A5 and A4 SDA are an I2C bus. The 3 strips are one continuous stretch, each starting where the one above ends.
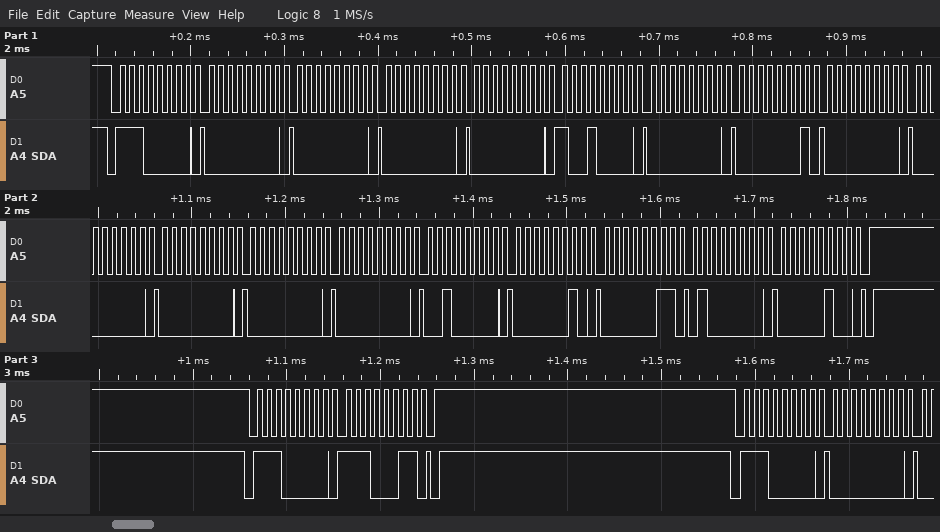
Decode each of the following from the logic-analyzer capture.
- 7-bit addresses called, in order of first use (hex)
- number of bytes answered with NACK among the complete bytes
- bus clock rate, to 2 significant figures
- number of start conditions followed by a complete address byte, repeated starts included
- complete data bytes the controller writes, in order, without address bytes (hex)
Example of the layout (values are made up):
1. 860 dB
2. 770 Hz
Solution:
1. 0x70
2. 0
3. 100 kHz
4. 3
5. 00 00 00 00 90 00 01 00 00 00 00 00 20 02 03 40 04 E3 00
